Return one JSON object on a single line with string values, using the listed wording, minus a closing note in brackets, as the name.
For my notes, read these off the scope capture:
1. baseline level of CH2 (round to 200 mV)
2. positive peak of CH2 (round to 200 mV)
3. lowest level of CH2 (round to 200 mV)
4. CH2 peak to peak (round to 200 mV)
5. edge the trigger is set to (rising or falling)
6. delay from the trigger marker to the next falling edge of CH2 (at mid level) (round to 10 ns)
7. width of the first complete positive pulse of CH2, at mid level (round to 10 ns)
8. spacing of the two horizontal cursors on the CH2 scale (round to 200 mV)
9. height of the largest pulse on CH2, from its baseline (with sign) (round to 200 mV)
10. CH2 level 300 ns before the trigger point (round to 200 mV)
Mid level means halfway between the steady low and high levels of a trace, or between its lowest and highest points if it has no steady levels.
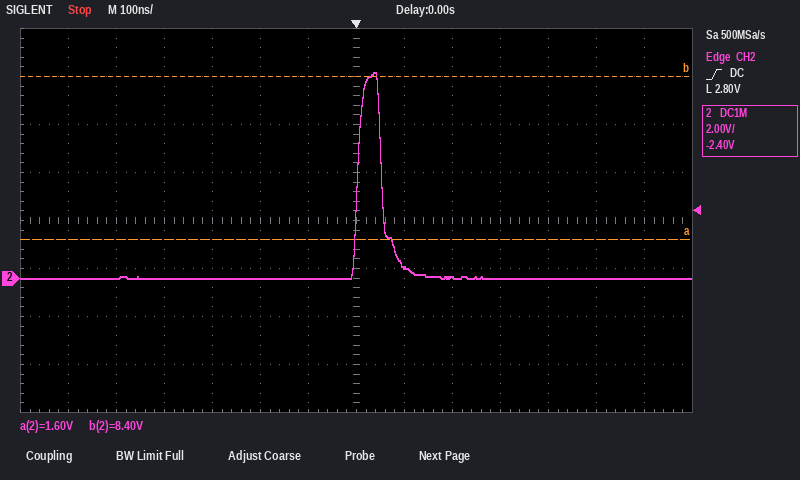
{"baseline level of CH2": "0.0 V", "positive peak of CH2": "8.6 V", "lowest level of CH2": "0.0 V", "CH2 peak to peak": "8.6 V", "edge the trigger is set to": "rising", "delay from the trigger marker to the next falling edge of CH2 (at mid level)": "50 ns", "width of the first complete positive pulse of CH2, at mid level": "50 ns", "spacing of the two horizontal cursors on the CH2 scale": "6.8 V", "height of the largest pulse on CH2, from its baseline (with sign)": "+8.6 V", "CH2 level 300 ns before the trigger point": "0.0 V"}
